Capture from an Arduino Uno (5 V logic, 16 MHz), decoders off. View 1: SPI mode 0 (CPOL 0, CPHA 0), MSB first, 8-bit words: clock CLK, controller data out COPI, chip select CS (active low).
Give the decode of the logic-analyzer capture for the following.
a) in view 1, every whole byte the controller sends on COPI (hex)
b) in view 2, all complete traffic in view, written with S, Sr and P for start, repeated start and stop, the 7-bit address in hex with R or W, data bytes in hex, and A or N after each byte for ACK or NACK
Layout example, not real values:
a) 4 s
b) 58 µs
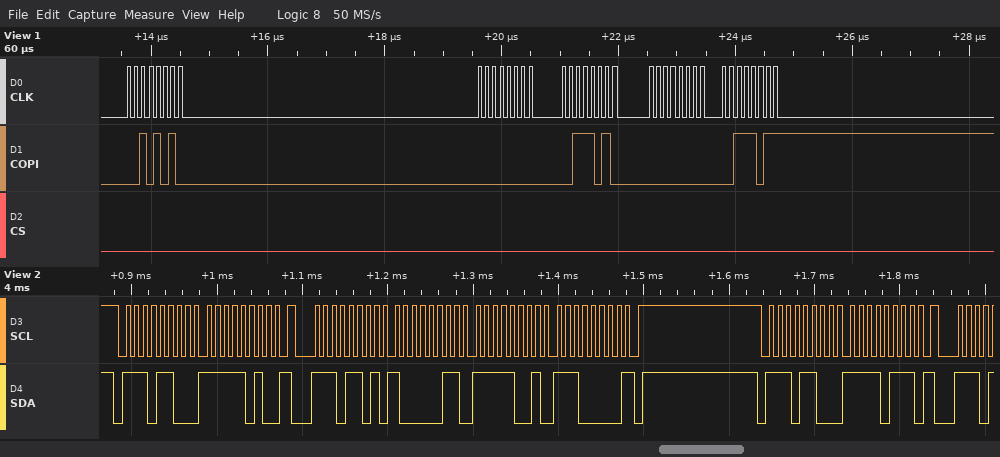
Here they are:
a) 2A 00 3A 00 3B
b) S 76W A FA A Sr 76R A 83 A F9 A E0 N P S 76W A F7 A
